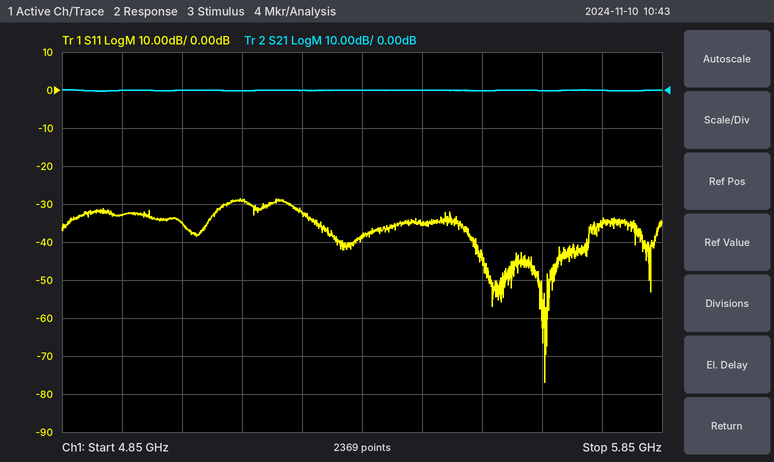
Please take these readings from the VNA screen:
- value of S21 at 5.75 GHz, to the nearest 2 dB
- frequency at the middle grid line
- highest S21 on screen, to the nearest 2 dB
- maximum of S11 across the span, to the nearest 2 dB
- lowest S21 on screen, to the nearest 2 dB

0 dB
5.35 GHz
0 dB
-28 dB
0 dB
